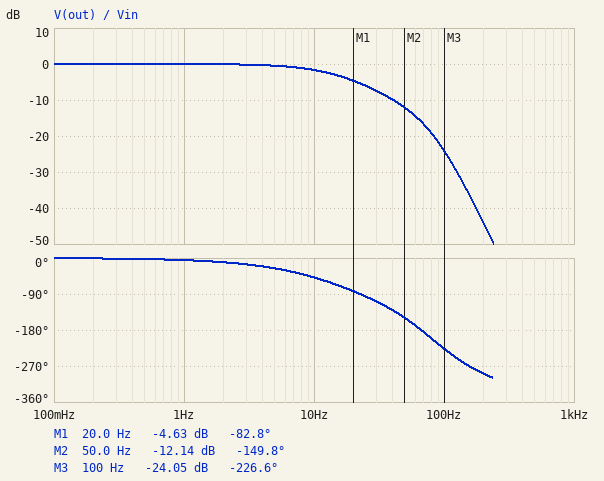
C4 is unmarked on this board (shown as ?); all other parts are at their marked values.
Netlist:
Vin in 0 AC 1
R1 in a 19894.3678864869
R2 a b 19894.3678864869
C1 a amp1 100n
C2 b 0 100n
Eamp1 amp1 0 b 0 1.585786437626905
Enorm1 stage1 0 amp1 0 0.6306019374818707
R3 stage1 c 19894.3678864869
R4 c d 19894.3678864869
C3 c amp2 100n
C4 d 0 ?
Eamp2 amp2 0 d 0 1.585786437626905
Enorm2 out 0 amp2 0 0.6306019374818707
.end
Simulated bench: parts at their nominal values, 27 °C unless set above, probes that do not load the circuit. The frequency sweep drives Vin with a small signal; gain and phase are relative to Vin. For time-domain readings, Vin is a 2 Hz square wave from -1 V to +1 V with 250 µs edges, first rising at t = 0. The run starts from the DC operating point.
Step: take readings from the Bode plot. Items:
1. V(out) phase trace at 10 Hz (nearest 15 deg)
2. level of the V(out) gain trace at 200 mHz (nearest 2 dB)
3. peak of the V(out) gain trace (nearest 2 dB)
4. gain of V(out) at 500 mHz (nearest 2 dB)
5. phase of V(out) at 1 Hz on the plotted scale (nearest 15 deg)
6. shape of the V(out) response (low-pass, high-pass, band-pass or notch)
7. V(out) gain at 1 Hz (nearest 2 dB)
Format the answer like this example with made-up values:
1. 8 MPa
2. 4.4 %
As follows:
1. -45 deg
2. 0 dB
3. 0 dB
4. 0 dB
5. 0 deg
6. low-pass
7. 0 dB
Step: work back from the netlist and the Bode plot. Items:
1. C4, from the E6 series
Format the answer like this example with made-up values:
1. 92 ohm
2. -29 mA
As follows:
1. 330 nF
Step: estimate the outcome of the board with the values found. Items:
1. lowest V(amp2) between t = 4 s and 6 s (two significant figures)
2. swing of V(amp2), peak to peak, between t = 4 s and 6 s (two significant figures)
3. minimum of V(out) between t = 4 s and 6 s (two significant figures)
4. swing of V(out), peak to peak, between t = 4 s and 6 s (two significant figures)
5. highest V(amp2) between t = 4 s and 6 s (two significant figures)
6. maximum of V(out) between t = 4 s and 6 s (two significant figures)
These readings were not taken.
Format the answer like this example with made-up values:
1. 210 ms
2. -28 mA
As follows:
1. -1.6 V
2. 3.2 V
3. -1.0 V
4. 2.0 V
5. 1.6 V
6. 1.0 V
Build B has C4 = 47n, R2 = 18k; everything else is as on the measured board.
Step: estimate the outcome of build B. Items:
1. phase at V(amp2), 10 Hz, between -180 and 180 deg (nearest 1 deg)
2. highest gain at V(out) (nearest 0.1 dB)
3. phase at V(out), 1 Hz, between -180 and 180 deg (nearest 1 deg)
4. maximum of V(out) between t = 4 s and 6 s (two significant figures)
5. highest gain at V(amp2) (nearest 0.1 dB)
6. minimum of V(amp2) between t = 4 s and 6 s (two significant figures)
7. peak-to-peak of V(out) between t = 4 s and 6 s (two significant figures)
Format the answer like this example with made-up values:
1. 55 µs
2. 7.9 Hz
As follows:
1. -12 deg
2. 1.5 dB
3. -1 deg
4. 1.5 V
5. 5.5 dB
6. -2.4 V
7. 3.0 V
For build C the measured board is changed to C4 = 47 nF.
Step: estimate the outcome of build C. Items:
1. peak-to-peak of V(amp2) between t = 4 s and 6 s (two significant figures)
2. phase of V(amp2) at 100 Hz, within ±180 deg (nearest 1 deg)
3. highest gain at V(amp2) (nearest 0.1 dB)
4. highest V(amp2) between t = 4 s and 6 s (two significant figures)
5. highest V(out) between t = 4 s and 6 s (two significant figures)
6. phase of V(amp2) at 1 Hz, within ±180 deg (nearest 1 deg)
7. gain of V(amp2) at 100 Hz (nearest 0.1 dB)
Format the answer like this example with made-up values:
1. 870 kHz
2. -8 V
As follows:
1. 4.5 V
2. -167 deg
3. 5.0 dB
4. 2.3 V
5. 1.4 V
6. -1 deg
7. 4.4 dB
